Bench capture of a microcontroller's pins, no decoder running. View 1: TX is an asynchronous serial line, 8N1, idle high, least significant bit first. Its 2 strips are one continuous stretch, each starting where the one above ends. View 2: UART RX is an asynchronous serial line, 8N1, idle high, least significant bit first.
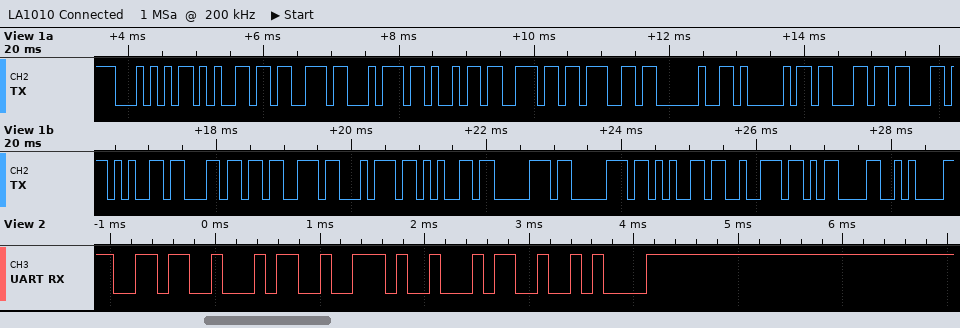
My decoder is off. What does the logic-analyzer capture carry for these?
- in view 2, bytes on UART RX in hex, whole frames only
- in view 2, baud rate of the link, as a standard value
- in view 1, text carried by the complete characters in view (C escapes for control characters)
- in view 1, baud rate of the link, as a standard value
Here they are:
0x36 0x34 0x2E 0x34 0x0A
9600 baud
"Testing Accelstepper\r\n"
9600 baud
